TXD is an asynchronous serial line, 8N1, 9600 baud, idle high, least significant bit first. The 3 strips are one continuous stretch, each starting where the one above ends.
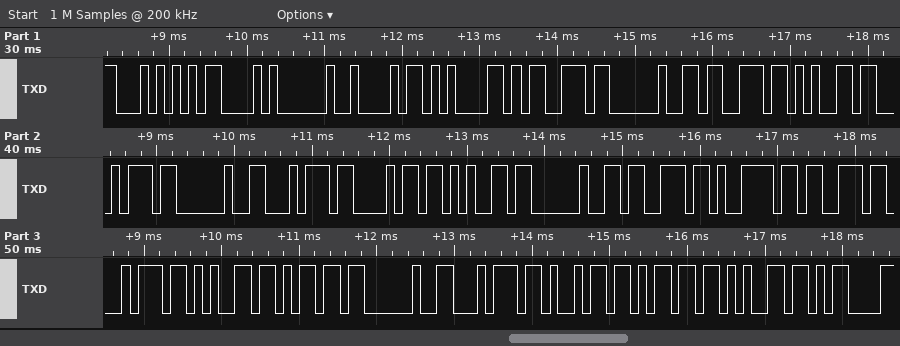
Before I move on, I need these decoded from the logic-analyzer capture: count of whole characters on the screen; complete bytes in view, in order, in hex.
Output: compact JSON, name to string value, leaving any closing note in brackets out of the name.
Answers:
{"count of whole characters on the screen": "27", "complete bytes in view, in order, in hex": "0x54 0x43 0x20 0x68 0x61 0x73 0x20 0x73 0x65 0x74 0x20 0x74 0x68 0x65 0x20 0x73 0x79 0x73 0x74 0x65 0x6D 0x20 0x74 0x69 0x6D 0x65 0x0D"}
